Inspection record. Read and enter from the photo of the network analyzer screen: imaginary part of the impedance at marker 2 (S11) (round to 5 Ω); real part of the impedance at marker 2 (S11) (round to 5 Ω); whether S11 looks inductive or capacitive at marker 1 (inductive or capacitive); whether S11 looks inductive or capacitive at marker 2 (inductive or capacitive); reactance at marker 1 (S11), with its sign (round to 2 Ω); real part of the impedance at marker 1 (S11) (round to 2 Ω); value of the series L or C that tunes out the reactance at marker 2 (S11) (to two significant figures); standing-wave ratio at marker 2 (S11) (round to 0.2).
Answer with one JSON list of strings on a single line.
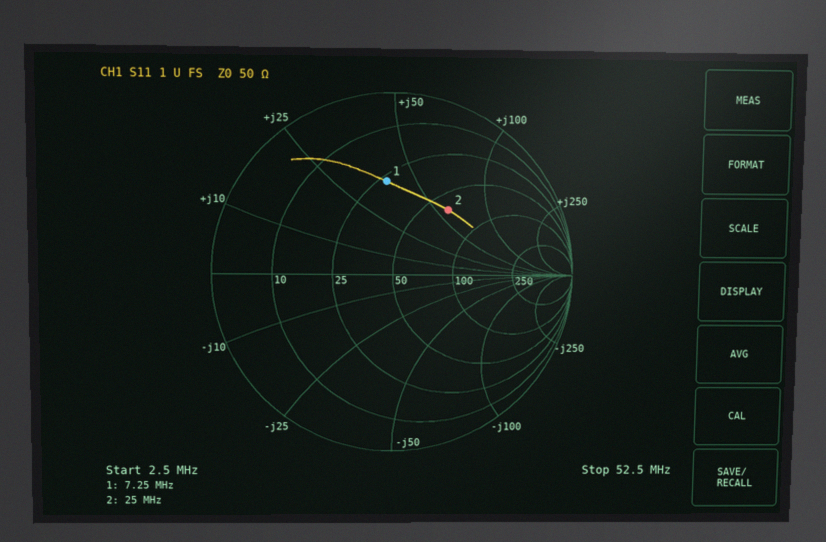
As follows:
["+60 Ω", "65 Ω", "inductive", "inductive", "+38 Ω", "28 Ω", "110 pF", "2.8"]
